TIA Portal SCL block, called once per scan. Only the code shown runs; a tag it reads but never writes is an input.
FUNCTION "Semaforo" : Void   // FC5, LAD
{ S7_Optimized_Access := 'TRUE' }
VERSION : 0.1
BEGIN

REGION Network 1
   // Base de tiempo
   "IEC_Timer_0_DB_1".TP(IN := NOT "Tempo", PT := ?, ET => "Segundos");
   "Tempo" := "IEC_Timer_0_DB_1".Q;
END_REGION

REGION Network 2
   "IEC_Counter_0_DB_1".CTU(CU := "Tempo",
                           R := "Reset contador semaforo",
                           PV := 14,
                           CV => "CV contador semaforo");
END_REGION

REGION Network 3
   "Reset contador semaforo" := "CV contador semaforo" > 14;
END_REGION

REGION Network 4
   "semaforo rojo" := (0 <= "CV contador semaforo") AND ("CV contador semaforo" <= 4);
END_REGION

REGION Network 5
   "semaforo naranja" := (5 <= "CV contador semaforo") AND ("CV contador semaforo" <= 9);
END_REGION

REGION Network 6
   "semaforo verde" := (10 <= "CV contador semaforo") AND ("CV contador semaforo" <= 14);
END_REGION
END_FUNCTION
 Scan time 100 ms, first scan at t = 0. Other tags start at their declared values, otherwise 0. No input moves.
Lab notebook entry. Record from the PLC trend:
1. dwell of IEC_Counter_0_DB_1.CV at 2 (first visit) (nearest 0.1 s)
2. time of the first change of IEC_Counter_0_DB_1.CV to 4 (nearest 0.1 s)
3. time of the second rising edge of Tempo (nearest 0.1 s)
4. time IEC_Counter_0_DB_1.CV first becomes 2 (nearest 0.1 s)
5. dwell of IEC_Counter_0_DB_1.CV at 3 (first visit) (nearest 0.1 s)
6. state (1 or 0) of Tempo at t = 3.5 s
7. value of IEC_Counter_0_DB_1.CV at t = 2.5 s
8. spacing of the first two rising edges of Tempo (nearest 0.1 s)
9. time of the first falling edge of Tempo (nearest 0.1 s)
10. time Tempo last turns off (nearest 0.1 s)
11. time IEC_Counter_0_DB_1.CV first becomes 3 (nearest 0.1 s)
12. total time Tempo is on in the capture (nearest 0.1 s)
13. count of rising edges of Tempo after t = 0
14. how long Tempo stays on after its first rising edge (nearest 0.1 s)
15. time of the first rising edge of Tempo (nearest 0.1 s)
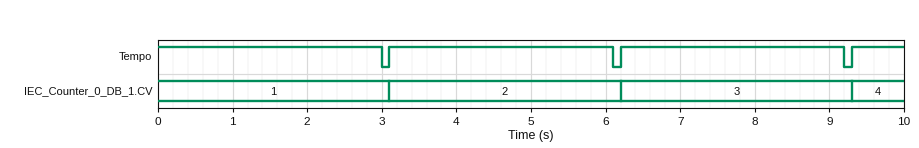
3.1 s
9.3 s
6.2 s
3.1 s
3.1 s
1
1
3.1 s
3.0 s
9.2 s
6.2 s
9.7 s
3
3.0 s
3.1 s
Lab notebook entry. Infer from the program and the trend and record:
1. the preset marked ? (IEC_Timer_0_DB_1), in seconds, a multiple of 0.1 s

3.0 s
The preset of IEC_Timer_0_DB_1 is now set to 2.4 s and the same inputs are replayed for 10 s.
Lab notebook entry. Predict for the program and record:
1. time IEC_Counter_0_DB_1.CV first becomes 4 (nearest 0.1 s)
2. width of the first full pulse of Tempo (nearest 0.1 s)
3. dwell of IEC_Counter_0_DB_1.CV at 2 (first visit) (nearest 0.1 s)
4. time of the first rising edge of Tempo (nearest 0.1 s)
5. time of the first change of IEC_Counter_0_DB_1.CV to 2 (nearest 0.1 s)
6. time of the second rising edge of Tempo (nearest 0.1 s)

7.5 s
2.4 s
2.5 s
2.5 s
2.5 s
5.0 s
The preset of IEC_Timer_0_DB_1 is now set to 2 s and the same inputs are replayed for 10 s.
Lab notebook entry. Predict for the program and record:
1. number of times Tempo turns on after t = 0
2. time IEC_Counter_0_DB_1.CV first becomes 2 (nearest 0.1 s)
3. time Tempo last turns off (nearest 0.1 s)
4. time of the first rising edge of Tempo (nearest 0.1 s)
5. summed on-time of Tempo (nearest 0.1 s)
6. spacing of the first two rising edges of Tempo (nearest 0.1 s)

4
2.1 s
8.3 s
2.1 s
9.6 s
2.1 s
